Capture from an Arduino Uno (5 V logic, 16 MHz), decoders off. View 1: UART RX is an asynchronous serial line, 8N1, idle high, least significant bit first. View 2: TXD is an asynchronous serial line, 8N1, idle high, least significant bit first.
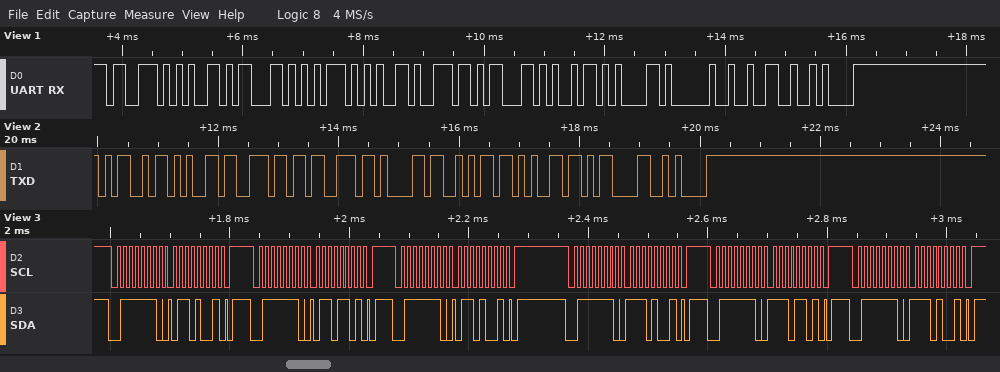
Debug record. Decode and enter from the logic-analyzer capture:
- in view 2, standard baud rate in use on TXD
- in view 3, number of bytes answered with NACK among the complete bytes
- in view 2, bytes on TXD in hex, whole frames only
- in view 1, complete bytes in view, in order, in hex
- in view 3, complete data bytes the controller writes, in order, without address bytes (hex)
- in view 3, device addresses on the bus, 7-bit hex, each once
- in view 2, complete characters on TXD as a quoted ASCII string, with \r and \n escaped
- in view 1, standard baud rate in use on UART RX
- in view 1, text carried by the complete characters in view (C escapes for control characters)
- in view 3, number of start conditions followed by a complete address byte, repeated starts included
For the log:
9600 baud
0
0x4D 0x65 0x6E 0x73 0x61 0x6A 0x65 0x0D 0x0A
73 65 63 75 65 6E 63 69 61 20 32 0A
69 6D 69 E9 ED E9
0x3F
"Mensaje\r\n"
9600 baud
"secuencia 2\n"
6
